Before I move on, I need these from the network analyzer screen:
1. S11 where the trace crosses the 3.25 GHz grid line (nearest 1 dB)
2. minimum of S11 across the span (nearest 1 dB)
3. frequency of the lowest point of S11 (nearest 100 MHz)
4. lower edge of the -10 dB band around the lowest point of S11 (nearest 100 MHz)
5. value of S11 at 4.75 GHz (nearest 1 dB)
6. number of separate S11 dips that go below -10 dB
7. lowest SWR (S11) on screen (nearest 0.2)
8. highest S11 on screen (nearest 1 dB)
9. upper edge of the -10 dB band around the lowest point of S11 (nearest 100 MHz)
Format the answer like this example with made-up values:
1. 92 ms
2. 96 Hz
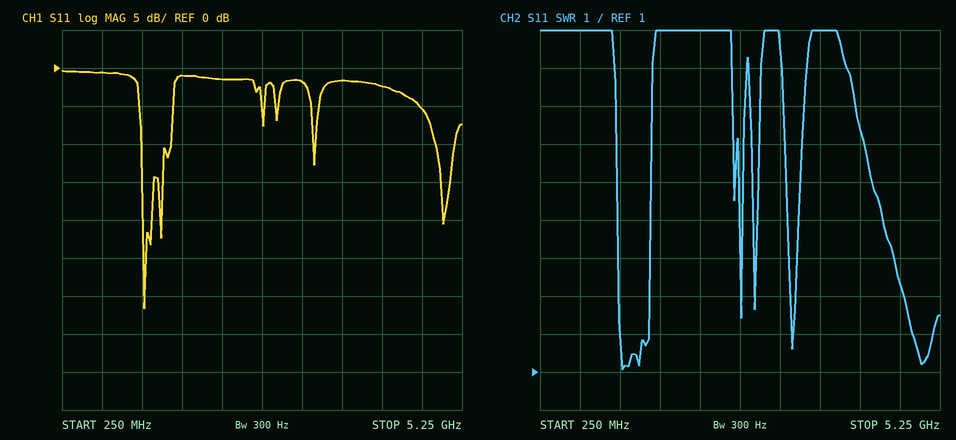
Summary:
1. -2 dB
2. -32 dB
3. 1.3 GHz
4. 1.2 GHz
5. -5 dB
6. 4
7. 1.0
8. 0 dB
9. 1.6 GHz
